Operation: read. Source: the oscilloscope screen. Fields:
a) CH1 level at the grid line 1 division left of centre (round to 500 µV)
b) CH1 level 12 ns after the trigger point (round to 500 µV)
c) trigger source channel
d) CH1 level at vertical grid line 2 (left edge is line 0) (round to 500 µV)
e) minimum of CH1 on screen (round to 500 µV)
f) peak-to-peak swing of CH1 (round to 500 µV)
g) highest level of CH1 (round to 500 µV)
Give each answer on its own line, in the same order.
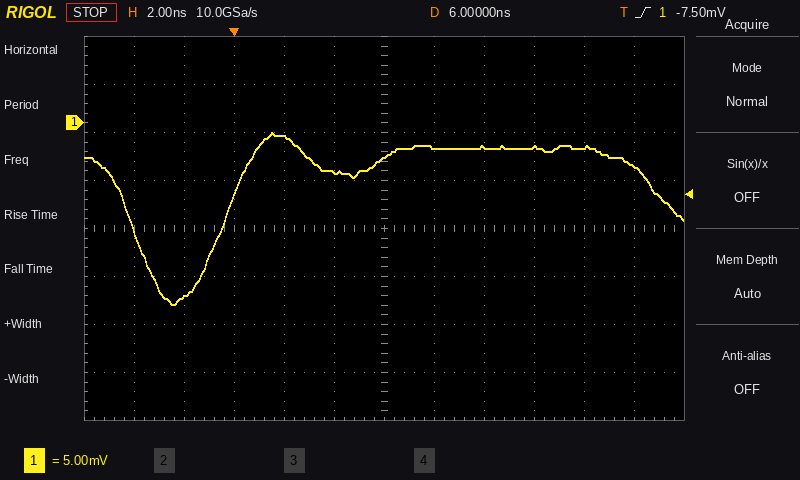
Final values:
-5.0 mV
-2.5 mV
CH1
-18.0 mV
-19.0 mV
18.0 mV
-1.0 mV
